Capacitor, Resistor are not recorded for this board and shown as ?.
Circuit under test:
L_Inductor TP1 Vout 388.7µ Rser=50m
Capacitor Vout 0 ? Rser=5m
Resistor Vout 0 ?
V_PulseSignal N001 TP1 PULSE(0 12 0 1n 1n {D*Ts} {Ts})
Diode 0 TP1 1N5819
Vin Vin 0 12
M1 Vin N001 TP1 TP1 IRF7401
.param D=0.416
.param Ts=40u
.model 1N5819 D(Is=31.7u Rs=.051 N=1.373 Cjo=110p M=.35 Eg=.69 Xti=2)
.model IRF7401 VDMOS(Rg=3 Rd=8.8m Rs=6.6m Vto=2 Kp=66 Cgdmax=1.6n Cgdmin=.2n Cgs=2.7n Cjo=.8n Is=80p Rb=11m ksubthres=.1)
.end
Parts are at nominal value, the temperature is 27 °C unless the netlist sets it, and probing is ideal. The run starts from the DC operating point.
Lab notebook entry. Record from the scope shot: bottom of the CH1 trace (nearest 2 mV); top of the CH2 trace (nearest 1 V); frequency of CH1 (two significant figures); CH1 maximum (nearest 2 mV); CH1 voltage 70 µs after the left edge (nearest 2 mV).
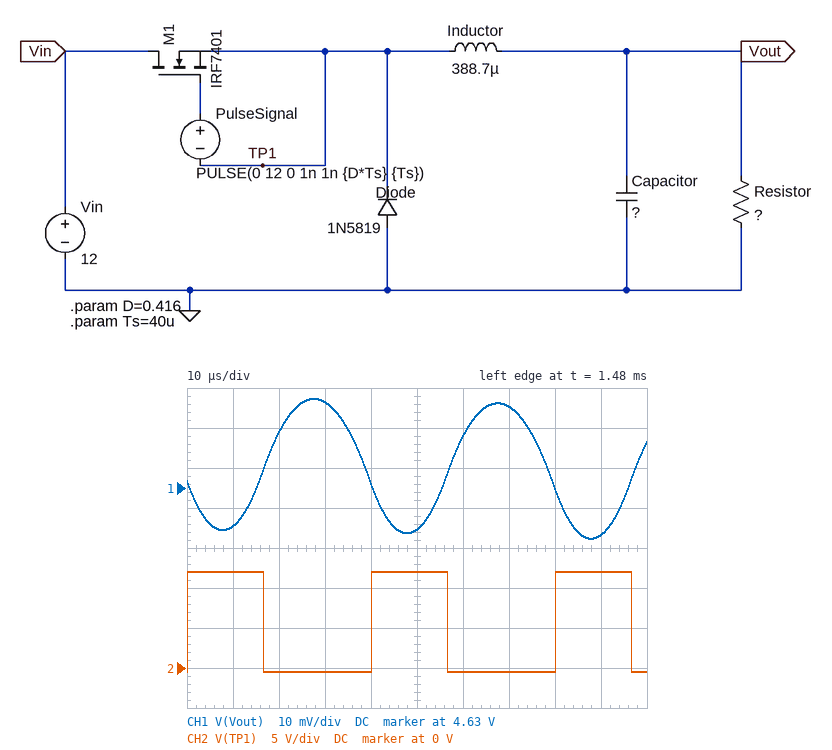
4.618 V
12 V
25 kHz
4.652 V
4.650 V
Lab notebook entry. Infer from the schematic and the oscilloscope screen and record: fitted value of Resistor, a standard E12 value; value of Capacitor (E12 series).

2.7 Ω
47 µF
